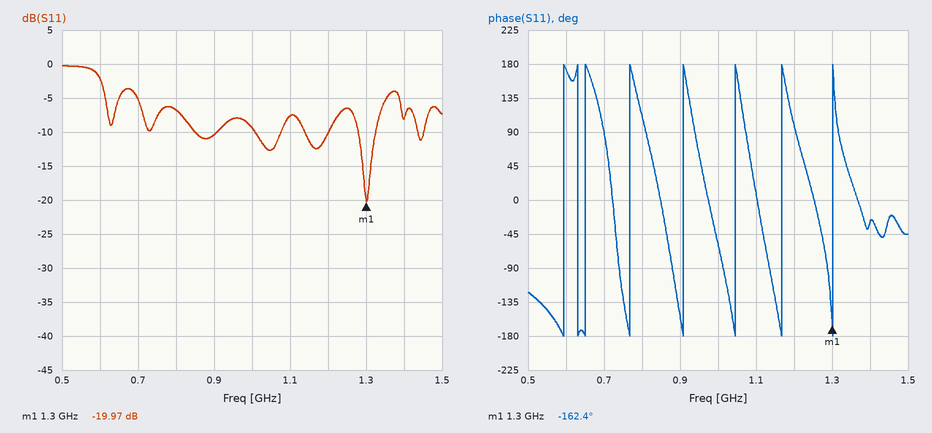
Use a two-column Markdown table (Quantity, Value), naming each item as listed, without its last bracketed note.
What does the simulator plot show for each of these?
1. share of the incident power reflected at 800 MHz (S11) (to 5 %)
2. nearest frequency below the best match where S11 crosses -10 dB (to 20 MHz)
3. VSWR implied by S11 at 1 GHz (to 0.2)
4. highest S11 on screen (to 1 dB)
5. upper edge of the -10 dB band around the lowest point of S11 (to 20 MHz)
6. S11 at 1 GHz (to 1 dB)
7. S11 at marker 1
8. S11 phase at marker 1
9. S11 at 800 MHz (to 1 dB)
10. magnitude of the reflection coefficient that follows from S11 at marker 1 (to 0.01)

| Quantity | Value |
|---|---|
| share of the incident power reflected at 800 MHz (S11) | 20 % |
| nearest frequency below the best match where S11 crosses -10 dB | 1.28 GHz |
| VSWR implied by S11 at 1 GHz | 2.0 |
| highest S11 on screen | 0 dB |
| upper edge of the -10 dB band around the lowest point of S11 | 1.32 GHz |
| S11 at 1 GHz | -9 dB |
| S11 at marker 1 | -19.97 dB |
| S11 phase at marker 1 | -162.4° |
| S11 at 800 MHz | -7 dB |
| magnitude of the reflection coefficient that follows from S11 at marker 1 | 0.10 |
